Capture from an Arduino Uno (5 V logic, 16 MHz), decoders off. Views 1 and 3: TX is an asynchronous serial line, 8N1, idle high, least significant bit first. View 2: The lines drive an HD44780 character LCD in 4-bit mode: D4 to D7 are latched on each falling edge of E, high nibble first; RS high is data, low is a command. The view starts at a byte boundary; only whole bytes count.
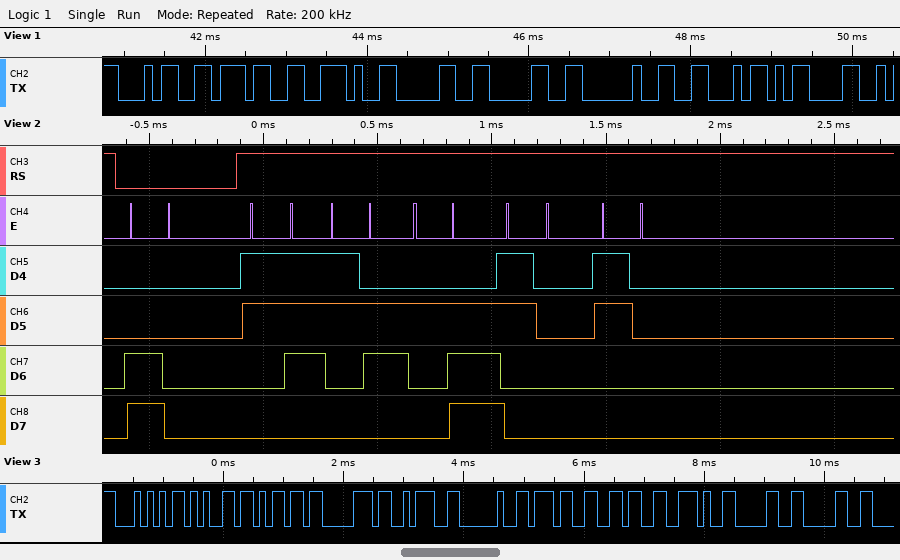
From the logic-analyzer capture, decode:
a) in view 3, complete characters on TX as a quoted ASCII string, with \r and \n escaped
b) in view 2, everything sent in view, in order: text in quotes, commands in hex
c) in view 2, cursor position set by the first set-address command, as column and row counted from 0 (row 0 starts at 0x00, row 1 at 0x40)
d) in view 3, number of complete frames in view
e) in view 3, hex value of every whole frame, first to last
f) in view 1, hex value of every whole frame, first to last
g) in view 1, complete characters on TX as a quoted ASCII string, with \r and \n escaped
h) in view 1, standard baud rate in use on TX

"Temp: 76.00"
0xC0 "76.00"
column 0, row 1
11
54 65 6D 70 3A 20 37 36 2E 30 30
0x34 0x37 0x2E 0x30 0x30 0x20 0x46 0x0D
"47.00 F\r"
9600 baud
